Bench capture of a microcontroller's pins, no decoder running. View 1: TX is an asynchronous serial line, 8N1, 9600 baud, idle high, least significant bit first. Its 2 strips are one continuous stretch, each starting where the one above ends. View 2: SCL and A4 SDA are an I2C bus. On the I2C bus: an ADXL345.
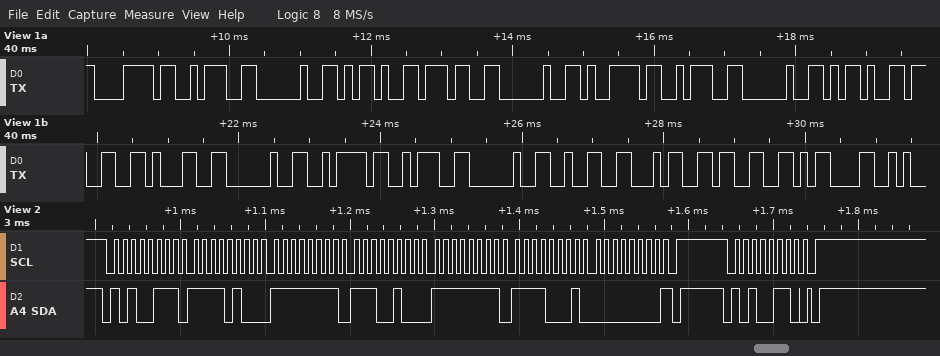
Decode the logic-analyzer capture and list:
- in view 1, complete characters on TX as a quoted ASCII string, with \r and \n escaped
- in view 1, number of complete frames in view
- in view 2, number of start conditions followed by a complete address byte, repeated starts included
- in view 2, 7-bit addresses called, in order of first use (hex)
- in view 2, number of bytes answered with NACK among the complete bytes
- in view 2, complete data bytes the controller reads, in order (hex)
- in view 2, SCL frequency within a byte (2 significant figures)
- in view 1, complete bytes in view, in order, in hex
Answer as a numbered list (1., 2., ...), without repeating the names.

1. "x: -7 y: -31 z: 243\r"
2. 20
3. 2
4. 0x53
5. 1
6. F4 FF E4 FF F1 00
7. 100 kHz
8. 78 3A 20 2D 37 20 79 3A 20 2D 33 31 20 7A 3A 20 32 34 33 0D
